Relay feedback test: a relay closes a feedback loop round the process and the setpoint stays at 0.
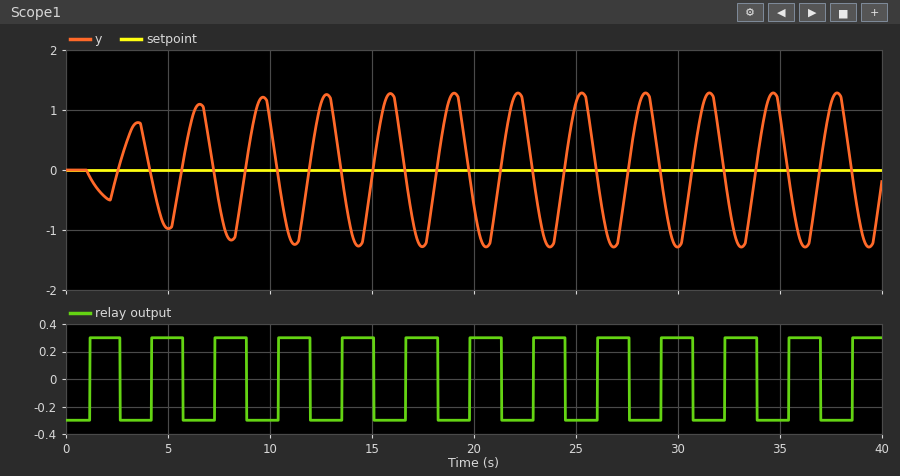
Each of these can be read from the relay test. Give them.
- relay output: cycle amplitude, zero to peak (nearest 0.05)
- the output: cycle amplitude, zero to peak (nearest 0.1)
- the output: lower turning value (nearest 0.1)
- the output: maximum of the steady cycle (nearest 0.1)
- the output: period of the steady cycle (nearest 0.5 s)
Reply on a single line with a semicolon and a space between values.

0.30; 1.3; -1.3; 1.3; 3.0 s
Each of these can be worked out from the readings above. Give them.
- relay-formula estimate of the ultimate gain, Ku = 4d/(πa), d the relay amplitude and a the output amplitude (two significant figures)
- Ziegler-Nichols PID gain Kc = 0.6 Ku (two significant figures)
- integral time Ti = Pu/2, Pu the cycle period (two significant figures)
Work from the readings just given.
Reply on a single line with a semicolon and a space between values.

0.29; 0.17; 1.5 s
